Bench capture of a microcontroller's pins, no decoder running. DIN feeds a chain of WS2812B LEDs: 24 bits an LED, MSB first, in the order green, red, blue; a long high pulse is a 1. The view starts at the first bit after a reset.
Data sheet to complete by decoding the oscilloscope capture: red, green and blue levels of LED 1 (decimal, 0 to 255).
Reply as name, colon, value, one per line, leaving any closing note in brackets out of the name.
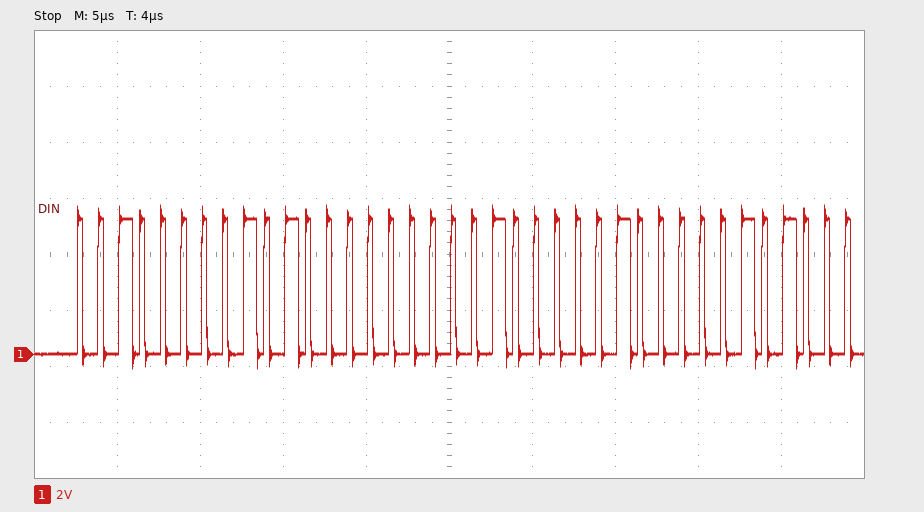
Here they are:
red, green and blue levels of LED 1: 160, 32, 8
